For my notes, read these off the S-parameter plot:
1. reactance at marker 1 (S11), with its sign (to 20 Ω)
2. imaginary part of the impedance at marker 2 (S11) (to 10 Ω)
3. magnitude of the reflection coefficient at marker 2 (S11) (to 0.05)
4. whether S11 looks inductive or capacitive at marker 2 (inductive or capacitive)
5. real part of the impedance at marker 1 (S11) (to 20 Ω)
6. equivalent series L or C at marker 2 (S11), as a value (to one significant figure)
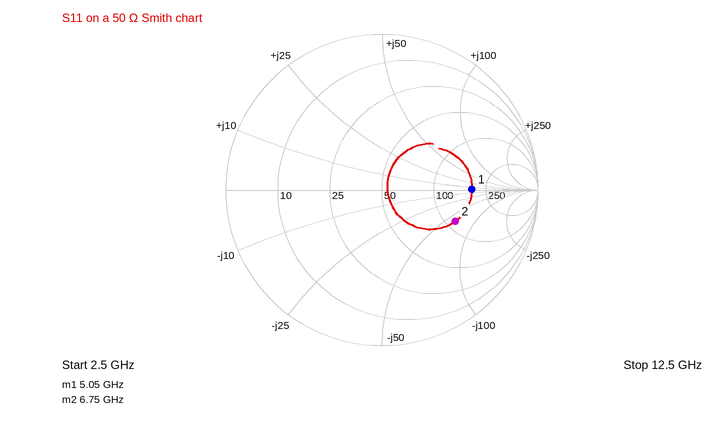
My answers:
0 Ω
-60 Ω
0.50
capacitive
180 Ω
400 fF
